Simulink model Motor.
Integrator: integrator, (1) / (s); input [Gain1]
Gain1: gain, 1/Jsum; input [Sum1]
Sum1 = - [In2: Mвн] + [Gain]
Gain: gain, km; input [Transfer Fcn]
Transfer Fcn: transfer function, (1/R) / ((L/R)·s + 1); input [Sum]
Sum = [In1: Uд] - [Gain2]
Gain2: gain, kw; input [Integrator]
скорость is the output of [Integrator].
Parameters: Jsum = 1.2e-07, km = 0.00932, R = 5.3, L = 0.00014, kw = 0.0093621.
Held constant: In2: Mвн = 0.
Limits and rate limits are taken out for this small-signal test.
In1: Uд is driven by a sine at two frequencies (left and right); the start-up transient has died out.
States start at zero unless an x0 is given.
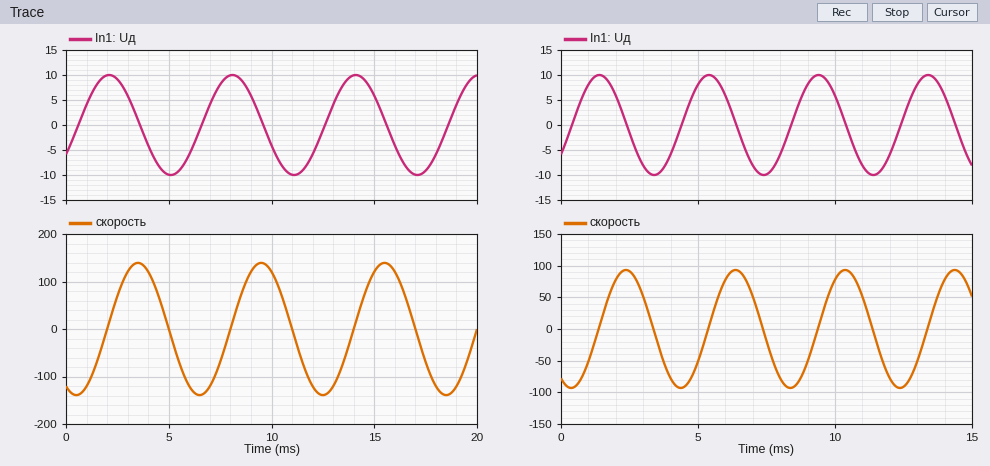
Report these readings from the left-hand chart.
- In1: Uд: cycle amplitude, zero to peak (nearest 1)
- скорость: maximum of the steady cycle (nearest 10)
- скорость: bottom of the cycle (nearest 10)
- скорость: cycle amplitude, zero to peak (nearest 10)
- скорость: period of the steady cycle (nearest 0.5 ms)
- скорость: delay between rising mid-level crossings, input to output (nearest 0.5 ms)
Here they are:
10
140
-140
140
6.0 ms
1.5 ms
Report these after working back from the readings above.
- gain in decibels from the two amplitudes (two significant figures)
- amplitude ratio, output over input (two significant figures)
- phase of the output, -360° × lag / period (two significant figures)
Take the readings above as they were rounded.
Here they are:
23 dB
14
-90°
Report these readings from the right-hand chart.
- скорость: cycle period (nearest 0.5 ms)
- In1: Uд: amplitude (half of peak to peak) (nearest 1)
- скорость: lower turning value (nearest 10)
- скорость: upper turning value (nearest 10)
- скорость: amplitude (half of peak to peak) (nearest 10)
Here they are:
4.0 ms
10
-90
90
90
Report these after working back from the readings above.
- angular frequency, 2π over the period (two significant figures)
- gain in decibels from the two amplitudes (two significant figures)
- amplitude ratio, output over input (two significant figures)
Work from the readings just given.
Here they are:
1.6 rad/ms
19 dB
9.0
